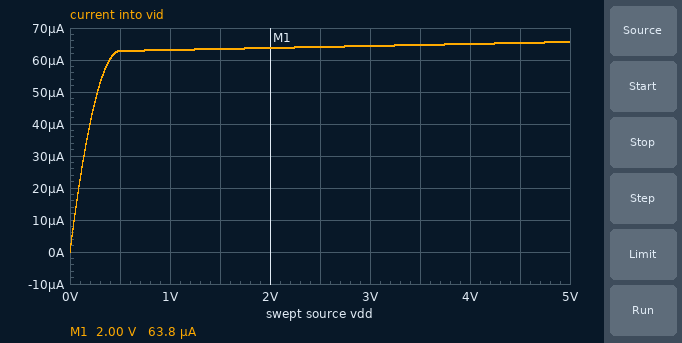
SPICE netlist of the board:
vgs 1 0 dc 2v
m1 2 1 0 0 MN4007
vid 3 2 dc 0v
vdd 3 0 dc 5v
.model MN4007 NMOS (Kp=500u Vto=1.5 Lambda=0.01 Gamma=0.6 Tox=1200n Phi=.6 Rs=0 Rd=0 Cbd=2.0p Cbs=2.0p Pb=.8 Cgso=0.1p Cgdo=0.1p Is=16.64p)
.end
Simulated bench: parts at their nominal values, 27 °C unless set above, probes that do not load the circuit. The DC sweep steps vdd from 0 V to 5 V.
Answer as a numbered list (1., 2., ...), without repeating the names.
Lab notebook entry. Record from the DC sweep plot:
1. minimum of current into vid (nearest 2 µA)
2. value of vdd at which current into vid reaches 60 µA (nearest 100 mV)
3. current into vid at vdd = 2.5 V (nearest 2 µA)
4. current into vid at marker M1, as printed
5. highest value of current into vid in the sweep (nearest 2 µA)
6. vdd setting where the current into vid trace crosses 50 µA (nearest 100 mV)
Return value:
1. 0 A
2. 400 mV
3. 64 µA
4. 63.8 µA
5. 66 µA
6. 300 mV
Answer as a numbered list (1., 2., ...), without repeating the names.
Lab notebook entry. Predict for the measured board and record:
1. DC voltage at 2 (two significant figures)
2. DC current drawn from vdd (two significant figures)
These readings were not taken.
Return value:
1. 5.0 V
2. 66 µA
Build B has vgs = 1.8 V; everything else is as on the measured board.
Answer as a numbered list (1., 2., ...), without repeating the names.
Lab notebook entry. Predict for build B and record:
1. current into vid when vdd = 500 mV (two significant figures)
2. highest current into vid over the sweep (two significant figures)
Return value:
1. 23 µA
2. 24 µA
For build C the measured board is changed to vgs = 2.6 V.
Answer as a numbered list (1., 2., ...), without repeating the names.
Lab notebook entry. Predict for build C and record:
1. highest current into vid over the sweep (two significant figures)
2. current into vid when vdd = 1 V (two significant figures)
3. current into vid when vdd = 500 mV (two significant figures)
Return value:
1. 320 µA
2. 300 µA
3. 210 µA
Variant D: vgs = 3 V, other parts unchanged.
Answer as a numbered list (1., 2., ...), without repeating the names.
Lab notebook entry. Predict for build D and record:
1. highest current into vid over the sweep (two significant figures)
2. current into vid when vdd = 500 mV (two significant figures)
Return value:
1. 590 µA
2. 310 µA
